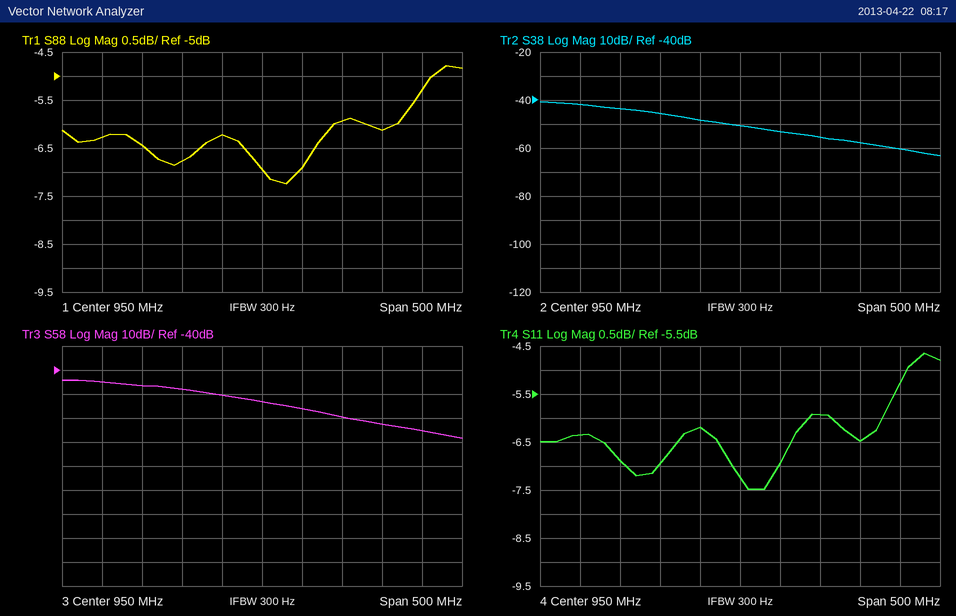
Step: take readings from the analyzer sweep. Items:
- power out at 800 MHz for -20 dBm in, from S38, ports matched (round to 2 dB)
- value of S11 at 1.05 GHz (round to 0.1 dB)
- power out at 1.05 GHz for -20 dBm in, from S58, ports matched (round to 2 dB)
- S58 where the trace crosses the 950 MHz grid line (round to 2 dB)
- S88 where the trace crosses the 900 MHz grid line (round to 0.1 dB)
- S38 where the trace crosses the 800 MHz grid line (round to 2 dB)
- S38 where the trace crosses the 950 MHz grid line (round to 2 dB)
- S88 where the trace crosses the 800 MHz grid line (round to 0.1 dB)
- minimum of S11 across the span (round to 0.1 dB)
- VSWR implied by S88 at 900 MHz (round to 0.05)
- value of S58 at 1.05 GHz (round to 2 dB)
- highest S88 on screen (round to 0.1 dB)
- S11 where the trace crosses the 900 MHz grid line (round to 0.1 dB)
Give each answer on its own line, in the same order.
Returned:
-64 dBm
-5.9 dB
-80 dBm
-54 dB
-6.2 dB
-44 dB
-50 dB
-6.4 dB
-7.5 dB
2.90
-60 dB
-4.8 dB
-6.2 dB
